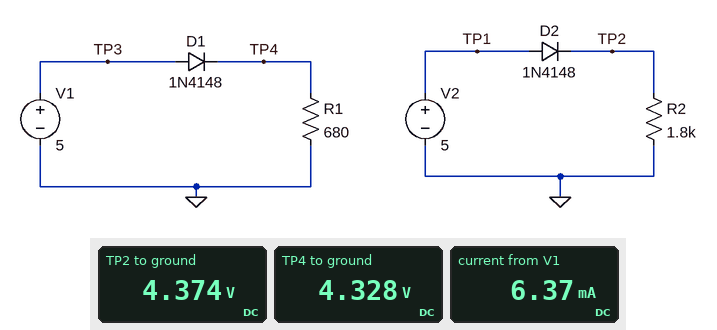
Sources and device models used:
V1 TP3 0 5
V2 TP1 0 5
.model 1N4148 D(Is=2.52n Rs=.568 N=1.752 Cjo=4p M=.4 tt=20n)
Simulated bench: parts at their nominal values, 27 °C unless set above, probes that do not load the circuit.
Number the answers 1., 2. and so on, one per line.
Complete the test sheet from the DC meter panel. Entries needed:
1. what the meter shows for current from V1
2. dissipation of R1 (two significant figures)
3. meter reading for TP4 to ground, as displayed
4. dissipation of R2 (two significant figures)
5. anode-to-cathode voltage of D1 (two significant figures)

1. 6.37 mA
2. 28 mW
3. 4.328 V
4. 11 mW
5. 670 mV
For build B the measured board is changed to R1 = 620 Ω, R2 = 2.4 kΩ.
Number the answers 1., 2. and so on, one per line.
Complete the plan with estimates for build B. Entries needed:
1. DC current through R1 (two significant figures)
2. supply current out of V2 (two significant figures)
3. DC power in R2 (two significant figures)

1. 7.0 mA
2. 1.8 mA
3. 8.0 mW
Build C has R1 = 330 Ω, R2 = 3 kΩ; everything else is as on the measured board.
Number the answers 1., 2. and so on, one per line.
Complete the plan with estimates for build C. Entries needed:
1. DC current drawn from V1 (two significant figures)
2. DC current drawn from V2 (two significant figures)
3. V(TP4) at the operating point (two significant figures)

1. 13 mA
2. 1.5 mA
3. 4.3 V
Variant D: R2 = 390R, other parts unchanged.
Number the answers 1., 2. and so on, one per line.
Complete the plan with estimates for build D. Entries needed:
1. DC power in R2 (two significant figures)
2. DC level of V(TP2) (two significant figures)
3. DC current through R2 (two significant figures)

1. 47 mW
2. 4.3 V
3. 11 mA
